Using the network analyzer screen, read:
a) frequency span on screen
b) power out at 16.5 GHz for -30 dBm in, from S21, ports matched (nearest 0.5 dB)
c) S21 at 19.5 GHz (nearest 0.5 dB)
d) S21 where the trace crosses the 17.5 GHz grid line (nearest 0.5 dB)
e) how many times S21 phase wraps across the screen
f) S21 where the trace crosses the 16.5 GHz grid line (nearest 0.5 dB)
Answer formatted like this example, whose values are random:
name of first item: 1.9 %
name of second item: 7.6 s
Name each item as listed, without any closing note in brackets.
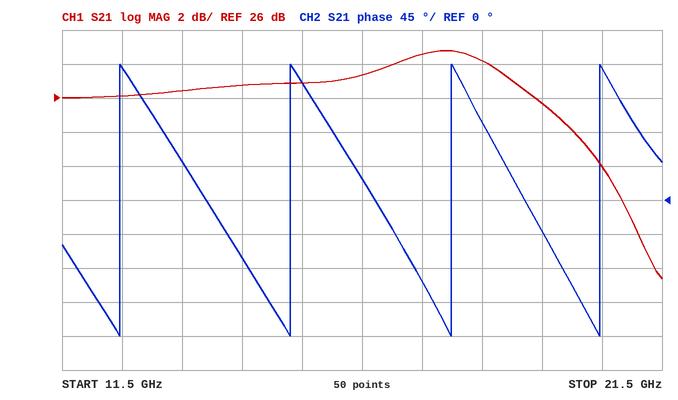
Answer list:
frequency span on screen: 10 GHz
power out at 16.5 GHz for -30 dBm in, from S21, ports matched: -2.5 dBm
S21 at 19.5 GHz: 25.5 dB
S21 where the trace crosses the 17.5 GHz grid line: 28.5 dB
how many times S21 phase wraps across the screen: 4
S21 where the trace crosses the 16.5 GHz grid line: 27.5 dB
